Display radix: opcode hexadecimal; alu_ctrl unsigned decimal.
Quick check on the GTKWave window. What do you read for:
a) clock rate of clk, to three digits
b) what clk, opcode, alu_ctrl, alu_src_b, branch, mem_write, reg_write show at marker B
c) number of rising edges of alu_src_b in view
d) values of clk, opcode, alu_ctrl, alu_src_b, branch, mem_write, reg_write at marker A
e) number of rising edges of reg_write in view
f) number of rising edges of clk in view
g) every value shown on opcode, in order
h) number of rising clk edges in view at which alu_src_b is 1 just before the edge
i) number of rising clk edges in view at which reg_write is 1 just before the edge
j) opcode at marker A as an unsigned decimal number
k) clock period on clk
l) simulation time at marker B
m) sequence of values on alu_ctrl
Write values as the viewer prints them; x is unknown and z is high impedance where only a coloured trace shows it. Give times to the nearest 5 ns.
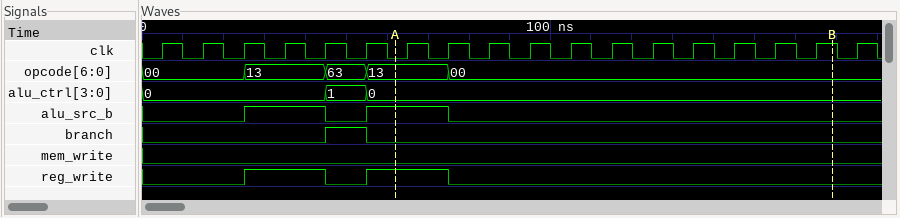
100 MHz
clk=1, opcode=00, alu_ctrl=0, alu_src_b=0, branch=0, mem_write=0, reg_write=0
2
clk=0, opcode=13, alu_ctrl=0, alu_src_b=1, branch=0, mem_write=0, reg_write=1
2
18
00, 13, 63, 13, 00
4
4
19
10 ns
170 ns
0, 1, 0
